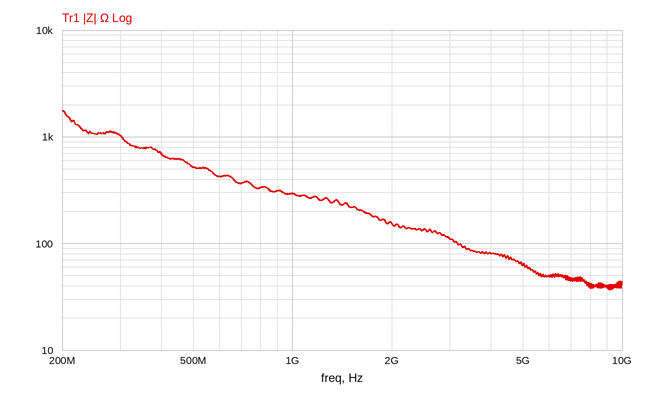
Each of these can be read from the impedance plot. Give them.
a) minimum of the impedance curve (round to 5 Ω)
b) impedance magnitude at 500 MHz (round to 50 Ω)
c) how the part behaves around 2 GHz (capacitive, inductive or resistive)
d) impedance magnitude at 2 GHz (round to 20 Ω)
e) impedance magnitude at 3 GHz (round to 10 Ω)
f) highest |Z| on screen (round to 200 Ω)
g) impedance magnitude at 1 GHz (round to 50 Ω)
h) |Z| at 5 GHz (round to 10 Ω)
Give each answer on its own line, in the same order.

35 Ω
500 Ω
capacitive
160 Ω
110 Ω
1.8 kΩ
300 Ω
60 Ω
